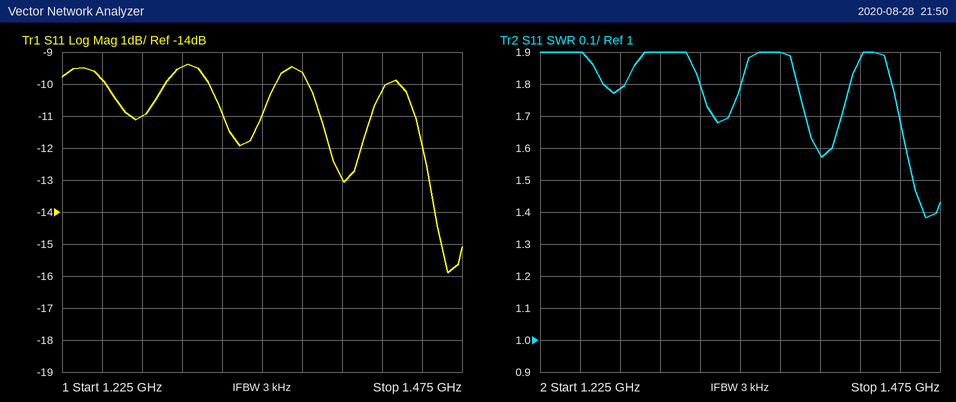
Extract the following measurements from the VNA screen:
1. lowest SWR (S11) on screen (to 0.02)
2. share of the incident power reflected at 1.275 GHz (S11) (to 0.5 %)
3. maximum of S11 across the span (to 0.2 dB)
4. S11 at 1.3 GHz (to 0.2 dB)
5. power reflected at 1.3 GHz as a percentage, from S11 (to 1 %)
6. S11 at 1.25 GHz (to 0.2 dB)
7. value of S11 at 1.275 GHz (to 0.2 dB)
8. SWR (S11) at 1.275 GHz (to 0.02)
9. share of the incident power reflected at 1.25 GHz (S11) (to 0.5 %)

1.38
8.0 %
-9.4 dB
-9.4 dB
11 %
-9.8 dB
-11.0 dB
1.78
10.5 %
